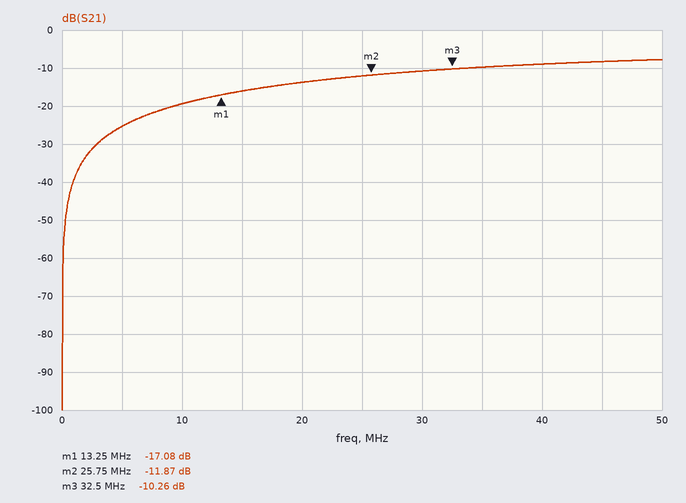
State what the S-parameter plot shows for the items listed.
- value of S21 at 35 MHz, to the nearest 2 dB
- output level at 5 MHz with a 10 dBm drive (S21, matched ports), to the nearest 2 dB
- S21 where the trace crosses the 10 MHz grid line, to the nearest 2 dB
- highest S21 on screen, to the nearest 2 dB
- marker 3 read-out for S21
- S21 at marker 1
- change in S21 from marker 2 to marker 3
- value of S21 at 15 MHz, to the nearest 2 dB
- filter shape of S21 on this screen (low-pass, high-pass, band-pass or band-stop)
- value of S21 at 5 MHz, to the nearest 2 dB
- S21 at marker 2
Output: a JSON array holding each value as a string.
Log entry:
["-10 dB", "-16 dBm", "-20 dB", "-8 dB", "-10.26 dB", "-17.08 dB", "1.61 dB", "-16 dB", "high-pass", "-26 dB", "-11.87 dB"]
